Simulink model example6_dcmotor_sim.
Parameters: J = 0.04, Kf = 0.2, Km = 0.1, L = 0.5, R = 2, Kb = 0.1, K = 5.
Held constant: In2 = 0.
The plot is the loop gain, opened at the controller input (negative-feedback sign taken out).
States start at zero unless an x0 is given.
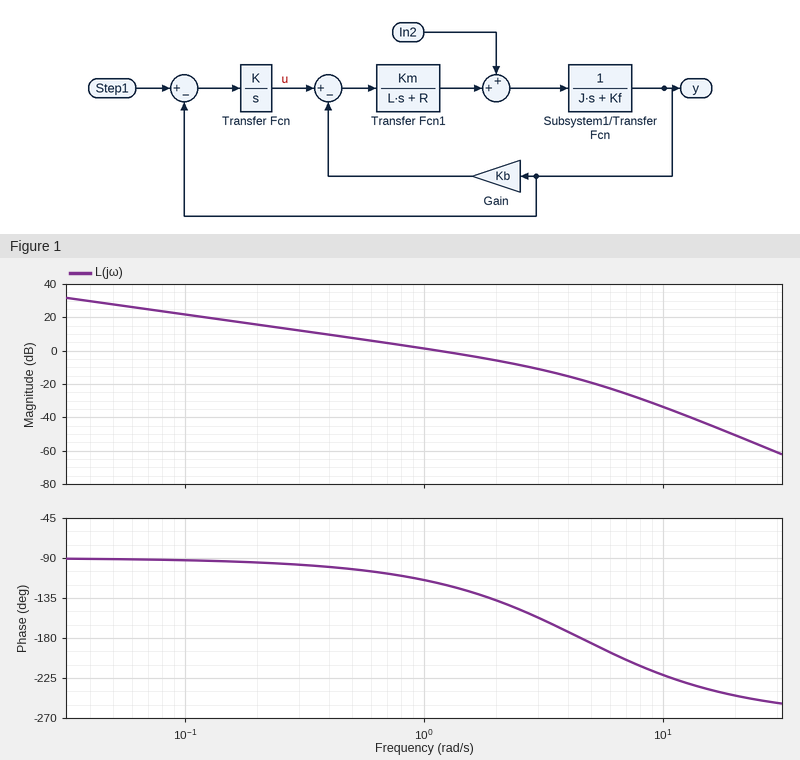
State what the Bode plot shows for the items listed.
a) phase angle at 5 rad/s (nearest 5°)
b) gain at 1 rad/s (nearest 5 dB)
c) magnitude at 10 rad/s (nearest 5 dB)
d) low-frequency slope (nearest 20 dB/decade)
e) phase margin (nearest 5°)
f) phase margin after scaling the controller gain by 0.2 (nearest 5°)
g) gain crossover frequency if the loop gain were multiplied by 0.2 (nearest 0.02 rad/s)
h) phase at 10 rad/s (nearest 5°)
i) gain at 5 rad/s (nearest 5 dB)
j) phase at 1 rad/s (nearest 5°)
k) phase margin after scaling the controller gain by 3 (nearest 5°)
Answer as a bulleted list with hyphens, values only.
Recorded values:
- -185°
- 0 dB
- -35 dB
- -20 dB/decade
- 60°
- 85°
- 0.24 rad/s
- -220°
- -20 dB
- -115°
- 30°
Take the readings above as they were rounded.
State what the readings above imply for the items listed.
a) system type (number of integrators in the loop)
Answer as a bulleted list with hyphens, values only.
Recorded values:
- 1
